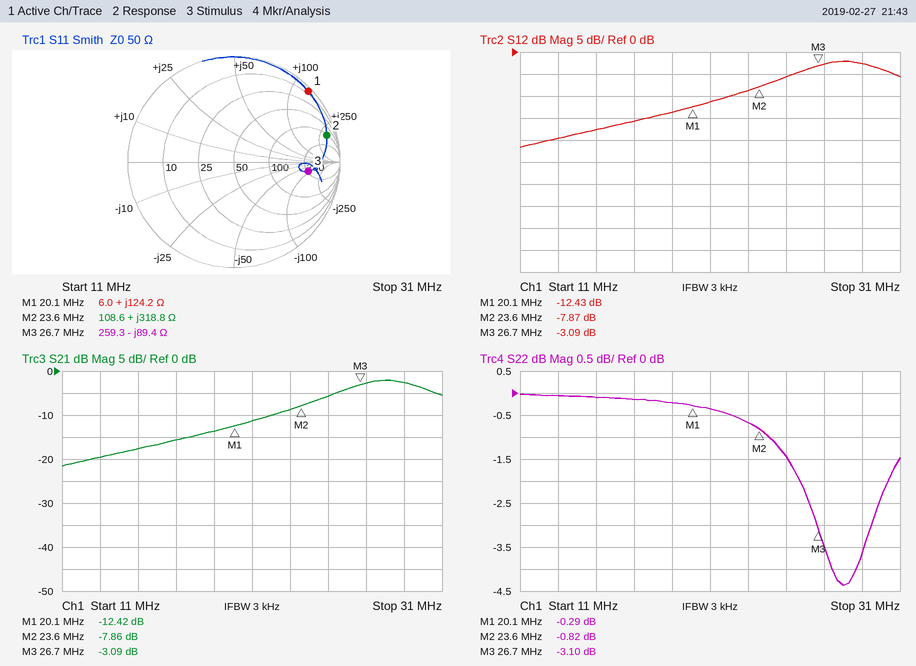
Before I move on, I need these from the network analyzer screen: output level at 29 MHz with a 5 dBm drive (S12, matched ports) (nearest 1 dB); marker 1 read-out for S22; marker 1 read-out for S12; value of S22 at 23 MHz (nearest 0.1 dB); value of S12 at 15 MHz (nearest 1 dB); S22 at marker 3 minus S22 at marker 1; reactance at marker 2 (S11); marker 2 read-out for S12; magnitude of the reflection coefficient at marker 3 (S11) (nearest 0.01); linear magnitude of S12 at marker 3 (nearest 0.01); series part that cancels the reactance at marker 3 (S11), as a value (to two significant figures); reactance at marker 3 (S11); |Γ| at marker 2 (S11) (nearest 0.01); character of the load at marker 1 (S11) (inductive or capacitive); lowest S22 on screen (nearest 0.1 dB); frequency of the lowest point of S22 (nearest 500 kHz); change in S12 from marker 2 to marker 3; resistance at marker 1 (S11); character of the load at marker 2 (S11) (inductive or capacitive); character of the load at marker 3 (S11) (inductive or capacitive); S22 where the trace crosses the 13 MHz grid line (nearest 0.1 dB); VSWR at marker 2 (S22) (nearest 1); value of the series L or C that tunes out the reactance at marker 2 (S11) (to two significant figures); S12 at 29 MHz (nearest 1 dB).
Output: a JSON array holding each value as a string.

["2 dBm", "-0.29 dB", "-12.43 dB", "-0.7 dB", "-18 dB", "-2.81 dB", "+318.8 Ω", "-7.87 dB", "0.71", "0.70", "530 nH", "-89.4 Ω", "0.91", "inductive", "-4.4 dB", "28.0 MHz", "4.78 dB", "6.0 Ω", "inductive", "capacitive", "-0.1 dB", "21", "21 pF", "-3 dB"]
